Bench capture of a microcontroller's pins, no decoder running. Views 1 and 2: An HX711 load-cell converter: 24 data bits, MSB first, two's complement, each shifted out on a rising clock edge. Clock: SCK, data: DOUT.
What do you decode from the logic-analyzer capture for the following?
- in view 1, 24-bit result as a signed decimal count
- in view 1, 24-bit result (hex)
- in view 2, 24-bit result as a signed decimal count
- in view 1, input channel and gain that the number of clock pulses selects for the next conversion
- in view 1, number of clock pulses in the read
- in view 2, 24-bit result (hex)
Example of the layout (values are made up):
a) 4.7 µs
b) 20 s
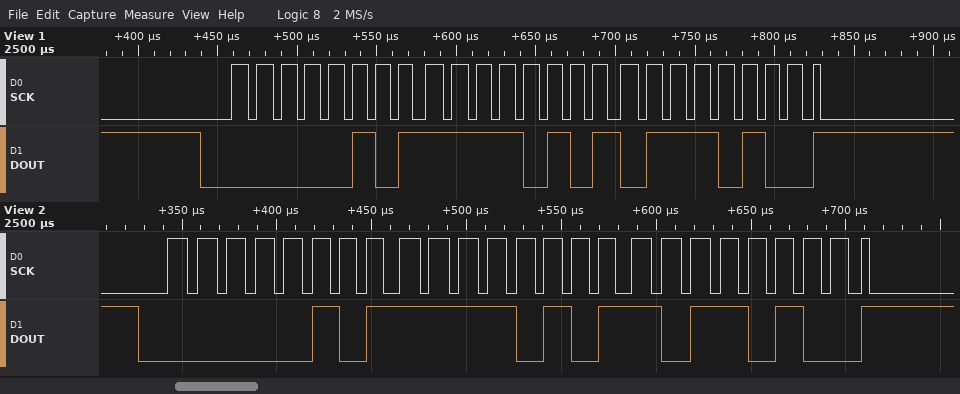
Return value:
a) 390516
b) 0x05F574
c) 390580
d) channel A, gain 128
e) 25
f) 0x05F5B4
